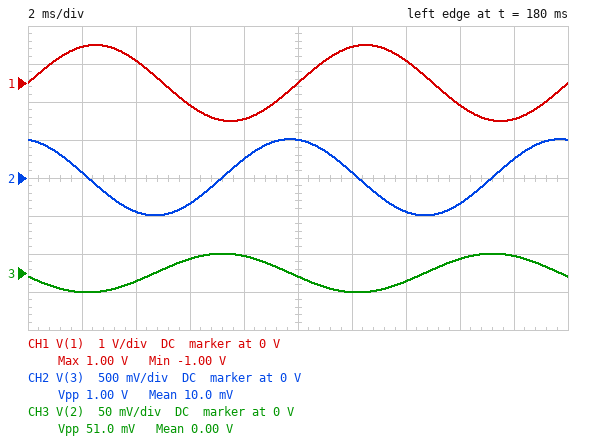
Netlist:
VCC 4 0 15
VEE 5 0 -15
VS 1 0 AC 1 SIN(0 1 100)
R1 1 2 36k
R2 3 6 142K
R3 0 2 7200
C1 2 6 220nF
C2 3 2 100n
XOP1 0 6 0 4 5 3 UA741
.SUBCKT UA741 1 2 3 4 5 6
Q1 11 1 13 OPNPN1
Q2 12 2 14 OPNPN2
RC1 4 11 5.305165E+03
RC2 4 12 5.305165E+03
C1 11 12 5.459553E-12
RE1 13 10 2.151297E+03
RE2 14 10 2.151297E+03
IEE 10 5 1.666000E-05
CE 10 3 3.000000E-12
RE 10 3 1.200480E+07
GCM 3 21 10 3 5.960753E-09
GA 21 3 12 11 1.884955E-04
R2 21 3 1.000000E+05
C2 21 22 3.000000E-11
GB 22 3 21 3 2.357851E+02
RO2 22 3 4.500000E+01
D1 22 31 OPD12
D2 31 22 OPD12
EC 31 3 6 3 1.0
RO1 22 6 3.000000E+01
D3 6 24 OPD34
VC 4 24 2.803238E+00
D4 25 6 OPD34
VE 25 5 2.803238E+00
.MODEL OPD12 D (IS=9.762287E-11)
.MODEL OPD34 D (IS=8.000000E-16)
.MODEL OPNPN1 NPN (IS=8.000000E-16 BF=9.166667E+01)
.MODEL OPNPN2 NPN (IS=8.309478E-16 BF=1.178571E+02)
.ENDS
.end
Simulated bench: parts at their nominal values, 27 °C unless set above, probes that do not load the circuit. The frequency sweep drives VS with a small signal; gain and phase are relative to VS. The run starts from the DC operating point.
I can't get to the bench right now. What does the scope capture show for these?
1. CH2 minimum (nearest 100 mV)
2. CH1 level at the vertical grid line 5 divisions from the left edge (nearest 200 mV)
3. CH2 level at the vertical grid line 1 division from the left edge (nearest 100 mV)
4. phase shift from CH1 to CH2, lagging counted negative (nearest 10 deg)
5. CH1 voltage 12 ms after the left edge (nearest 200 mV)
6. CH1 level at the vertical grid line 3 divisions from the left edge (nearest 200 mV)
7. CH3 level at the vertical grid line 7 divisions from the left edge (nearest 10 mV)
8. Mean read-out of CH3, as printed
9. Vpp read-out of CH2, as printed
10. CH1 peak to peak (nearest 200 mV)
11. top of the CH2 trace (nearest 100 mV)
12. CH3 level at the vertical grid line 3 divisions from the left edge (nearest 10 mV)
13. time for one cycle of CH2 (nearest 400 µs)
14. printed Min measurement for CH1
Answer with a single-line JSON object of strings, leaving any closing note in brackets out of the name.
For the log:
{"CH2 minimum": "-500 mV", "CH1 level at the vertical grid line 5 divisions from the left edge": "0 V", "CH2 level at the vertical grid line 1 division from the left edge": "100 mV", "phase shift from CH1 to CH2, lagging counted negative": "100 deg", "CH1 voltage 12 ms after the left edge": "1.0 V", "CH1 level at the vertical grid line 3 divisions from the left edge": "-600 mV", "CH3 level at the vertical grid line 7 divisions from the left edge": "-10 mV", "Mean read-out of CH3, as printed": "0.00 V", "Vpp read-out of CH2, as printed": "1.00 V", "CH1 peak to peak": "2.0 V", "top of the CH2 trace": "500 mV", "CH3 level at the vertical grid line 3 divisions from the left edge": "20 mV", "time for one cycle of CH2": "10.0 ms", "printed Min measurement for CH1": "-1.00 V"}
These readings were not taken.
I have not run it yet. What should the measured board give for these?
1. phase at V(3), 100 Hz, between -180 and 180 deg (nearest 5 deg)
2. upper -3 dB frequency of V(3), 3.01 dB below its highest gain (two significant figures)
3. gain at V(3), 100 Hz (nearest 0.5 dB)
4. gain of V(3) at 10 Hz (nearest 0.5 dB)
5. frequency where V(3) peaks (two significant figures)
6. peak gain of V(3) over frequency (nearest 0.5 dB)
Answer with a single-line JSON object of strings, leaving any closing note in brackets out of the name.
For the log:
{"phase at V(3), 100 Hz, between -180 and 180 deg": "100 deg", "upper -3 dB frequency of V(3), 3.01 dB below its highest gain": "46 Hz", "gain at V(3), 100 Hz": "-6.0 dB", "gain of V(3) at 10 Hz": "-9.0 dB", "frequency where V(3) peaks": "37 Hz", "peak gain of V(3) over frequency": "8.5 dB"}
